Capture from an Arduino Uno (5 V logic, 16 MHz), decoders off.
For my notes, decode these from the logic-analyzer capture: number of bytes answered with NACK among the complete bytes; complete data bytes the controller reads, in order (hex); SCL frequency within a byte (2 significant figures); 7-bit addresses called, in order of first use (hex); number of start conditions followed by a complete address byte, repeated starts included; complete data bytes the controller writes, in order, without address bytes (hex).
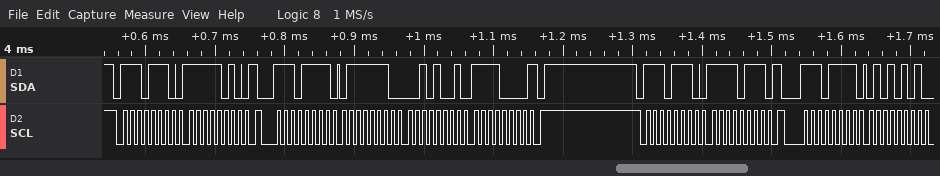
1
7E 29 F0 55
100 kHz
0x77
4
FA F7
